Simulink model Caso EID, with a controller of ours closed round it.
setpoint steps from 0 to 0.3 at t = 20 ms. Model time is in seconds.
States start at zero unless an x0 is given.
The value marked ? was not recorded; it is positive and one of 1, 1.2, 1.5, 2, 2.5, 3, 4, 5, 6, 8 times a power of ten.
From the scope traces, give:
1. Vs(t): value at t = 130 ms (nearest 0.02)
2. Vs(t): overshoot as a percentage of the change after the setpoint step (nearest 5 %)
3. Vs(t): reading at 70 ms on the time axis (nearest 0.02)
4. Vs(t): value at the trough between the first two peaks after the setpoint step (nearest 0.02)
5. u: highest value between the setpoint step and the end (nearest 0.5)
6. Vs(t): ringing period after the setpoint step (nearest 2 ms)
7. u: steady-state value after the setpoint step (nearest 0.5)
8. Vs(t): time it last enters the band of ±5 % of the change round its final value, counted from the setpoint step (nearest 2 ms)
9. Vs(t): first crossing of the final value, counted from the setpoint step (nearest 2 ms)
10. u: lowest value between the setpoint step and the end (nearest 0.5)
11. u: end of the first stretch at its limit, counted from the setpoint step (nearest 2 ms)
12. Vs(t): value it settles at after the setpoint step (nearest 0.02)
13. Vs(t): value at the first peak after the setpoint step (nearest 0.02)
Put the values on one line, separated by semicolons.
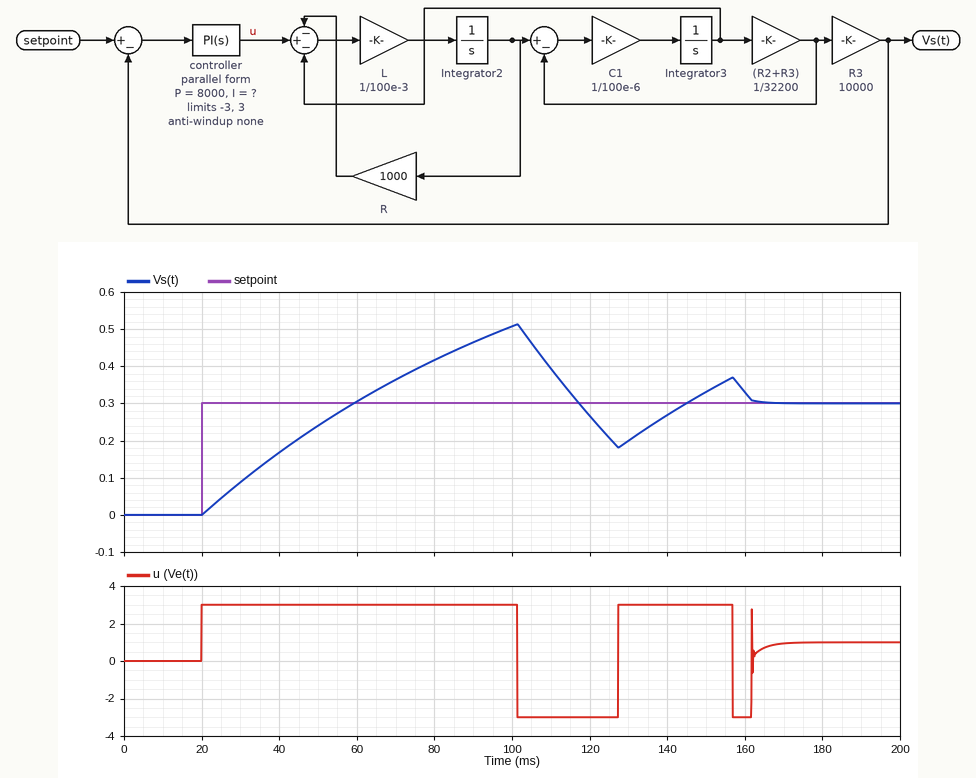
0.20; 70 %; 0.36; 0.18; 3.0; 56 ms; 1.0; 142 ms; 40 ms; -3.0; 82 ms; 0.30; 0.52
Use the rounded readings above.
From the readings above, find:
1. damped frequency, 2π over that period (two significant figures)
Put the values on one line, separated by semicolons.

0.11 rad/ms
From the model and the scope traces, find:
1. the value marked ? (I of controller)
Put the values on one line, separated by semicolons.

2.5e+06
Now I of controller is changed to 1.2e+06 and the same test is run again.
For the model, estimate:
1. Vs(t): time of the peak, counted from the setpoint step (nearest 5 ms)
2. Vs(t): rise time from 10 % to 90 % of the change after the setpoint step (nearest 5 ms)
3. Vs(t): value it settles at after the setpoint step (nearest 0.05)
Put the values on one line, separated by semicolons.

80 ms; 30 ms; 0.30
